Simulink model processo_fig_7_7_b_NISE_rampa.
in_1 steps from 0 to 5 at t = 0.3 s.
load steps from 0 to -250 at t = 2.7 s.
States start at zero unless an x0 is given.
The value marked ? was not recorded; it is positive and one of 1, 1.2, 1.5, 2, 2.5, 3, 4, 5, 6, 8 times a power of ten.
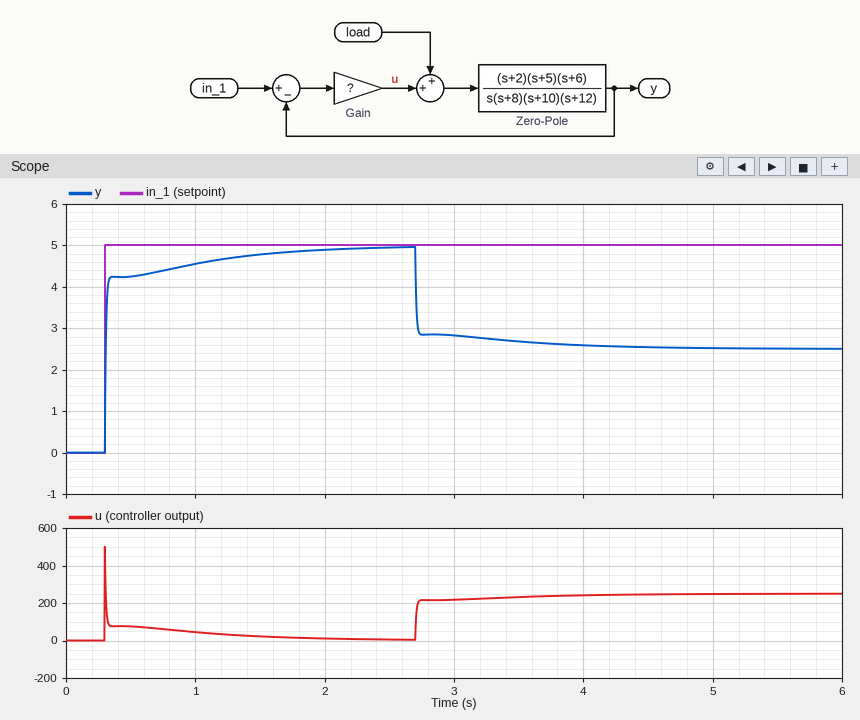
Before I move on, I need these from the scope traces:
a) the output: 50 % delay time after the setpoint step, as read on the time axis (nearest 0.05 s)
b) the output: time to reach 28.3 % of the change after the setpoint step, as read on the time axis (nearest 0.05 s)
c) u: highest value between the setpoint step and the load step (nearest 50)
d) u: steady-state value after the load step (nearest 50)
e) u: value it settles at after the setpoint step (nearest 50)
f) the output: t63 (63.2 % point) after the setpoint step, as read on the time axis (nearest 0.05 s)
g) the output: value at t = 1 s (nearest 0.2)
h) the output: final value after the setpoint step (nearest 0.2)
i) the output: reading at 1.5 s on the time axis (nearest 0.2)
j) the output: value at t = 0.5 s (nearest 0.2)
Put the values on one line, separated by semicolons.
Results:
0.30 s; 0.30 s; 500; 250; 0; 0.30 s; 4.6; 5.0; 4.8; 4.2
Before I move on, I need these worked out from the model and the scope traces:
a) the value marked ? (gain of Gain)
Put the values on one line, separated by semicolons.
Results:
100
